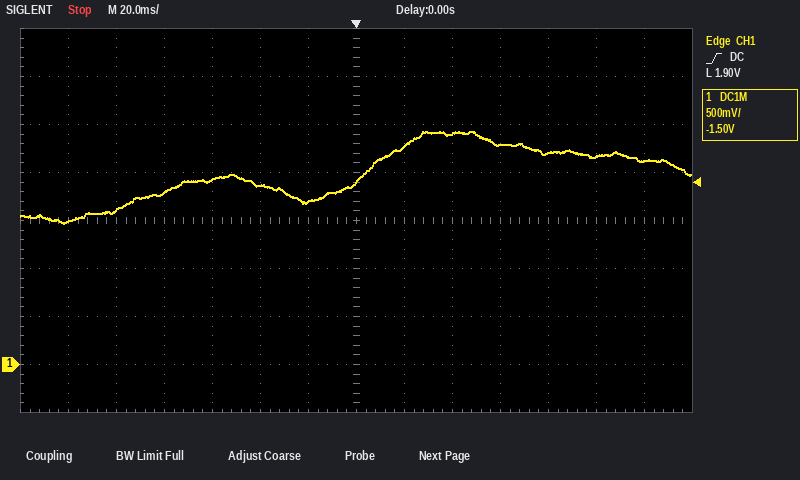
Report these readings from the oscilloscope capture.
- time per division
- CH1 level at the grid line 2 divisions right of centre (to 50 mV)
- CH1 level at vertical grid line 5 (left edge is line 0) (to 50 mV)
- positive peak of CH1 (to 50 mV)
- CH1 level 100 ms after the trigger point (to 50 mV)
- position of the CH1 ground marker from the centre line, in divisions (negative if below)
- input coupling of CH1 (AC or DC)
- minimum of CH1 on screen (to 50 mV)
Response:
20 ms
2.40 V
1.85 V
2.45 V
2.15 V
-3.0 div
DC
1.45 V
